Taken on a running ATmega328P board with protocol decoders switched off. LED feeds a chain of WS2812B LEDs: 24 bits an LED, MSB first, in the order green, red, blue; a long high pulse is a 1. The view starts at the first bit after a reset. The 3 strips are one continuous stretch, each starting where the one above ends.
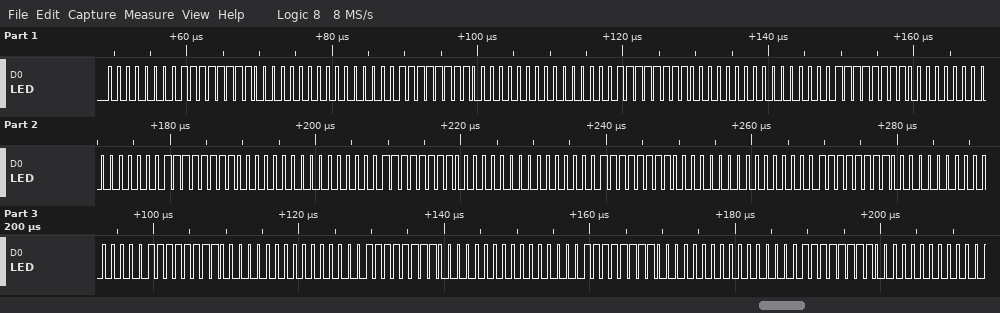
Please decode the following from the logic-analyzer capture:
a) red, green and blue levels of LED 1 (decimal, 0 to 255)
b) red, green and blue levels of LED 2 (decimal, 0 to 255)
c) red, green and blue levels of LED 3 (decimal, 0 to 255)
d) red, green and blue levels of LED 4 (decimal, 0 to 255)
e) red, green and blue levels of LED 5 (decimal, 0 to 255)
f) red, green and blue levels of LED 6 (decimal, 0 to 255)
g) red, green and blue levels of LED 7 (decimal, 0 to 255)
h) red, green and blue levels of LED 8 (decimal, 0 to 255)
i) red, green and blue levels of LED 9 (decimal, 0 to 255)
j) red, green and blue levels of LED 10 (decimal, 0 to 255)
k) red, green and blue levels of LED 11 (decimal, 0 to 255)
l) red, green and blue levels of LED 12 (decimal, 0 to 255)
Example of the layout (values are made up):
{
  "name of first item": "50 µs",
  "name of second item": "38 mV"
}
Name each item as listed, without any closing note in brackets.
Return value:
{
  "red, green and blue levels of LED 1": "255, 0, 0",
  "red, green and blue levels of LED 2": "255, 0, 0",
  "red, green and blue levels of LED 3": "255, 0, 0",
  "red, green and blue levels of LED 4": "255, 0, 0",
  "red, green and blue levels of LED 5": "255, 0, 0",
  "red, green and blue levels of LED 6": "255, 0, 0",
  "red, green and blue levels of LED 7": "255, 0, 0",
  "red, green and blue levels of LED 8": "255, 0, 0",
  "red, green and blue levels of LED 9": "255, 0, 0",
  "red, green and blue levels of LED 10": "255, 0, 0",
  "red, green and blue levels of LED 11": "255, 0, 0",
  "red, green and blue levels of LED 12": "255, 0, 0"
}
